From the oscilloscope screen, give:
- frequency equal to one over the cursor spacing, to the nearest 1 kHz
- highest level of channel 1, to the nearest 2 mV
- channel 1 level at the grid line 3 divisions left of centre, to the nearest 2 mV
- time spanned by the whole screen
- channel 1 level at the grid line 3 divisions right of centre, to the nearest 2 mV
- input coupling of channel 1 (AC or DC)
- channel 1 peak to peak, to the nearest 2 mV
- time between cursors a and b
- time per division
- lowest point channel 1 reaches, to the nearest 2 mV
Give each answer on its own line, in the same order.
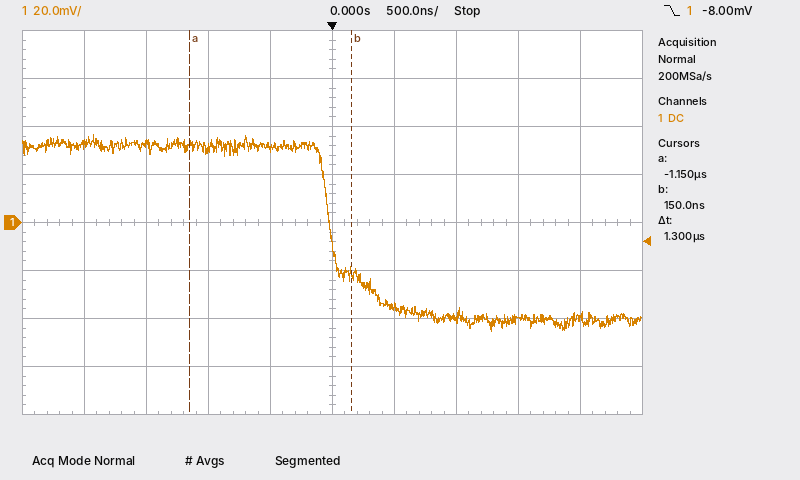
769 kHz
36 mV
32 mV
5 µs
-40 mV
DC
82 mV
1.3 µs
500 ns
-46 mV
